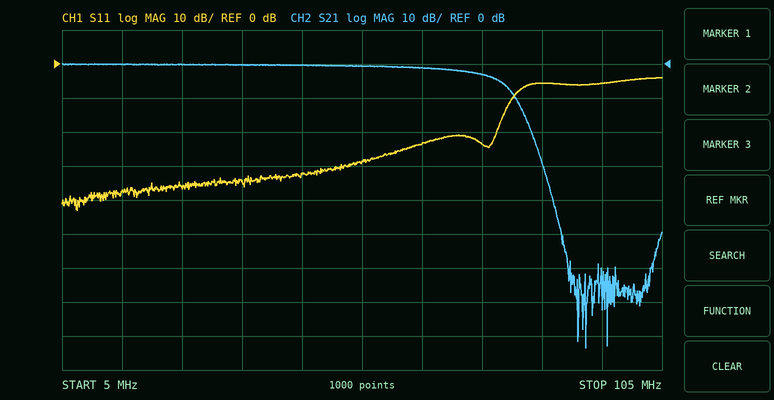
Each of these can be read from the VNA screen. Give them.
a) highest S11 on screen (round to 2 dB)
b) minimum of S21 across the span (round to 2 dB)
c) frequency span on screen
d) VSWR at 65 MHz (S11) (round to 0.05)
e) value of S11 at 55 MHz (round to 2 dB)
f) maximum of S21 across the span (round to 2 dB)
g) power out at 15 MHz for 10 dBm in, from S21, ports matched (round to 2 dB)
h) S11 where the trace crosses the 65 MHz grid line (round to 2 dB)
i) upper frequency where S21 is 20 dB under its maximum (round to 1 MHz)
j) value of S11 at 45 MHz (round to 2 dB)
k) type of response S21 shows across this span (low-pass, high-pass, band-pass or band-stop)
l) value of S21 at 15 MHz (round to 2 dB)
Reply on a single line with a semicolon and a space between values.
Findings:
-4 dB; -84 dB; 100 MHz; 1.15; -28 dB; 0 dB; 10 dBm; -24 dB; 83 MHz; -32 dB; low-pass; 0 dB
